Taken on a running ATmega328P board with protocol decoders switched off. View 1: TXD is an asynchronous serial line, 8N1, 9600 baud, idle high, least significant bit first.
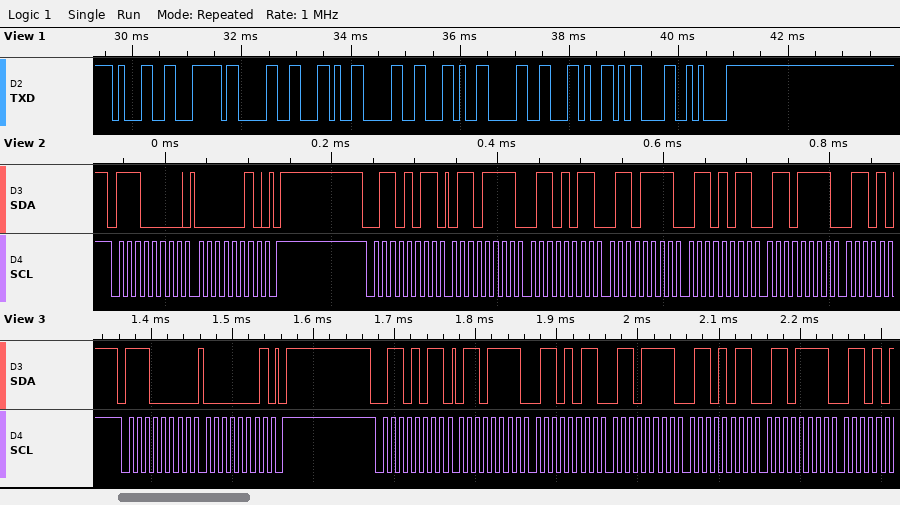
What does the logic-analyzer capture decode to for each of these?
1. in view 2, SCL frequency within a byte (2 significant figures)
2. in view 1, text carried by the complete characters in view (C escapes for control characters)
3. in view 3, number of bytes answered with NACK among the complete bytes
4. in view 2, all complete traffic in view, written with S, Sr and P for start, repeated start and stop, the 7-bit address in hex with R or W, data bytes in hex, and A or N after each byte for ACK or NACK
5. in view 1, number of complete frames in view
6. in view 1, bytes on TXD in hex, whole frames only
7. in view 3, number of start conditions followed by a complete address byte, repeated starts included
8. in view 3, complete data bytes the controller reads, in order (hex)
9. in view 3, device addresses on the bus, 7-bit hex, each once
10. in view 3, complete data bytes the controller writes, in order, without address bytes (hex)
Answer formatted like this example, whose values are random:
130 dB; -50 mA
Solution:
100 kHz; "1|0,0,0,\r\n"; 0; S 70W A 02 A P S 35R A 6F A 6B A 6F A 6B A 6F A; 10; 31 7C 30 2C 30 2C 30 2C 0D 0A; 2; 6F 6B 6F 6B 6F; 0x70 0x35; 01
